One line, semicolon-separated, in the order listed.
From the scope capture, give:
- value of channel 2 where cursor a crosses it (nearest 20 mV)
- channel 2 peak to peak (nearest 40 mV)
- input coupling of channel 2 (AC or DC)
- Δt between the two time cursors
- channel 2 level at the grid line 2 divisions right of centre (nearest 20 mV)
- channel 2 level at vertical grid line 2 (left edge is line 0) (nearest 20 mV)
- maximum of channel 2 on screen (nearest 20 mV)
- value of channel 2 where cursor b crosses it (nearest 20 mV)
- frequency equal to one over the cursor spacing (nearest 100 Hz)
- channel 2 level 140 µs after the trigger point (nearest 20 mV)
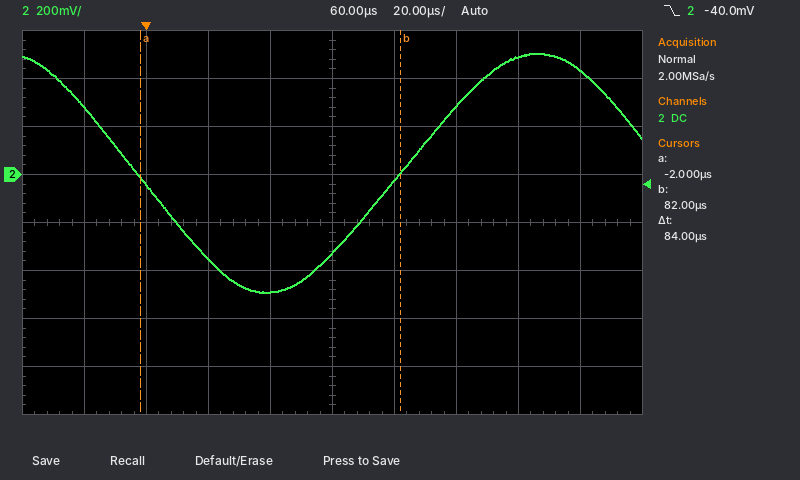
-20 mV; 1.00 V; DC; 84 µs; 280 mV; -40 mV; 500 mV; 0 mV; 11.9 kHz; 440 mV
